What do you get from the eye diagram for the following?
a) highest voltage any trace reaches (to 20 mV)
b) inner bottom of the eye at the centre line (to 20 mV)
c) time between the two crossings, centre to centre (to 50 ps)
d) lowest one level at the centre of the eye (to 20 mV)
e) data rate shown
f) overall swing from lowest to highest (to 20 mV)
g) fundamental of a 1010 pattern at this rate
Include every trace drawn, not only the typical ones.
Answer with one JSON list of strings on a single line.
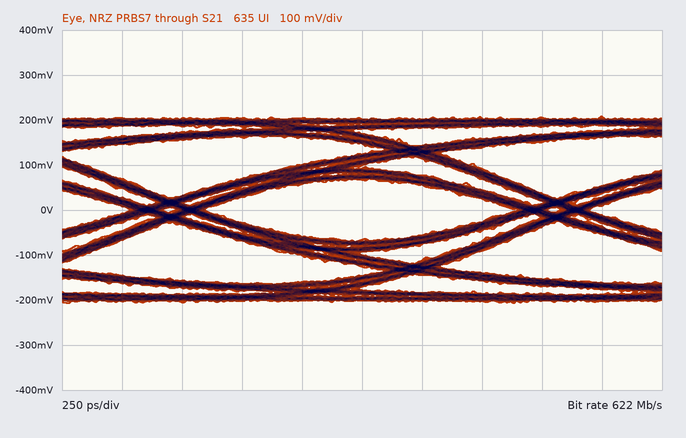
["200 mV", "-60 mV", "1.60 ns", "60 mV", "622 Mb/s", "420 mV", "311 MHz"]
